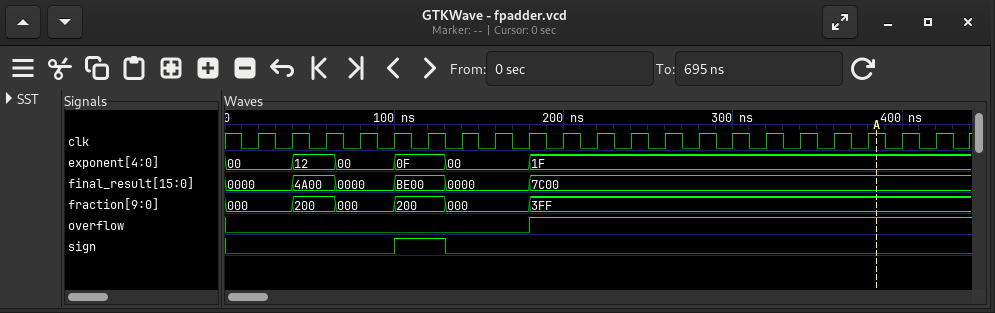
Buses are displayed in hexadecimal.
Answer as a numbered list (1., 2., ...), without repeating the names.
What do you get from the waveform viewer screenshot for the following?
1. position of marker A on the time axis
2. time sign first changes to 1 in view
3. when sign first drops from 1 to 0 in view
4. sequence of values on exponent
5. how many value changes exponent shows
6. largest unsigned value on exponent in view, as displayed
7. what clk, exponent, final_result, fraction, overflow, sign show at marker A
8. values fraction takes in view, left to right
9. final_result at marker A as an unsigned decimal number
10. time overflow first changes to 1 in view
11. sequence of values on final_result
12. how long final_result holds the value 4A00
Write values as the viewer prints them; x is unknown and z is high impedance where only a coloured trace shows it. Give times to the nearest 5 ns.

1. 385 ns
2. 100 ns
3. 130 ns
4. 00, 12, 00, 0F, 00, 1F
5. 5
6. 1F
7. clk=1, exponent=1F, final_result=7C00, fraction=3FF, overflow=1, sign=0
8. 000, 200, 000, 200, 000, 3FF
9. 31744
10. 180 ns
11. 0000, 4A00, 0000, BE00, 0000, 7C00
12. 25 ns
